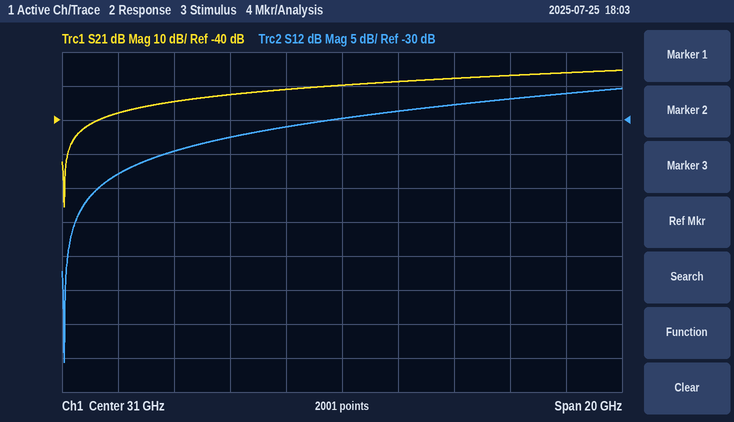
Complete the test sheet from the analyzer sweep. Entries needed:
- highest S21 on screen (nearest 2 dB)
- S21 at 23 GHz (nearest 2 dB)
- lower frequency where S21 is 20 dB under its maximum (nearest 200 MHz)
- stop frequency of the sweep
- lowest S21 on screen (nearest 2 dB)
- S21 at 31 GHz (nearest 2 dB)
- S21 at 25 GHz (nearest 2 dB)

-26 dB
-38 dB
21.4 GHz
41 GHz
-66 dB
-30 dB
-34 dB
